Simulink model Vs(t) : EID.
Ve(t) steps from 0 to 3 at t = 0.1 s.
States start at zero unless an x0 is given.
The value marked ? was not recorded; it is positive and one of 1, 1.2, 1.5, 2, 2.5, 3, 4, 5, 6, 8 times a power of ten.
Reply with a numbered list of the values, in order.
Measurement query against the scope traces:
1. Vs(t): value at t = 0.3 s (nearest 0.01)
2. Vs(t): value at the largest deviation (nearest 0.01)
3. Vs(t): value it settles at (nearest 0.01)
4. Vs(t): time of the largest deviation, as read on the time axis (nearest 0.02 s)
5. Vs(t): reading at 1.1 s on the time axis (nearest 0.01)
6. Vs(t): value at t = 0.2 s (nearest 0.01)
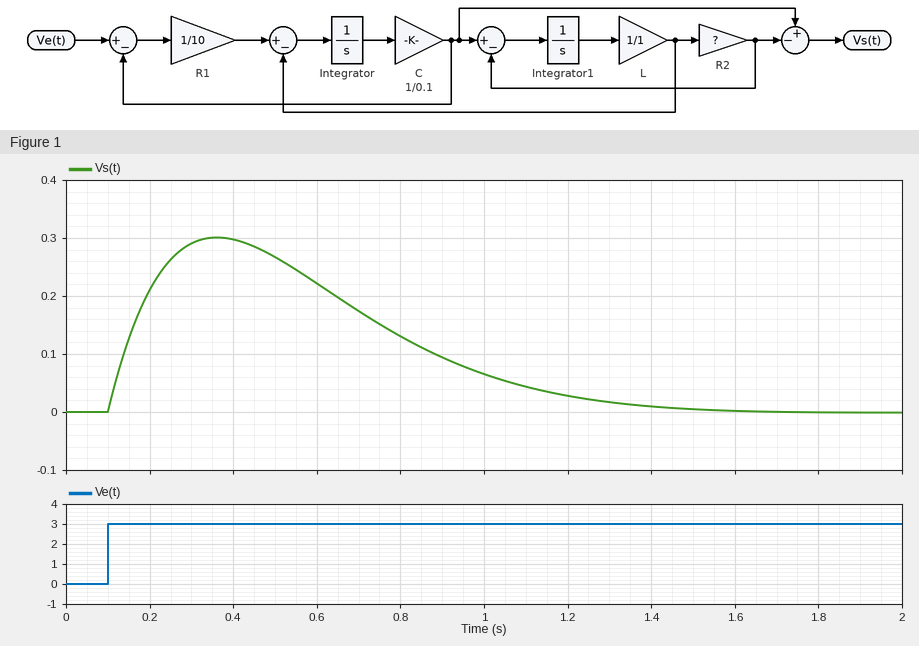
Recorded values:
1. 0.29
2. 0.30
3. 0.00
4. 0.36 s
5. 0.04
6. 0.21
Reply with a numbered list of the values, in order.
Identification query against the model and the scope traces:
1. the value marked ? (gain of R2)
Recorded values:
1. 6
